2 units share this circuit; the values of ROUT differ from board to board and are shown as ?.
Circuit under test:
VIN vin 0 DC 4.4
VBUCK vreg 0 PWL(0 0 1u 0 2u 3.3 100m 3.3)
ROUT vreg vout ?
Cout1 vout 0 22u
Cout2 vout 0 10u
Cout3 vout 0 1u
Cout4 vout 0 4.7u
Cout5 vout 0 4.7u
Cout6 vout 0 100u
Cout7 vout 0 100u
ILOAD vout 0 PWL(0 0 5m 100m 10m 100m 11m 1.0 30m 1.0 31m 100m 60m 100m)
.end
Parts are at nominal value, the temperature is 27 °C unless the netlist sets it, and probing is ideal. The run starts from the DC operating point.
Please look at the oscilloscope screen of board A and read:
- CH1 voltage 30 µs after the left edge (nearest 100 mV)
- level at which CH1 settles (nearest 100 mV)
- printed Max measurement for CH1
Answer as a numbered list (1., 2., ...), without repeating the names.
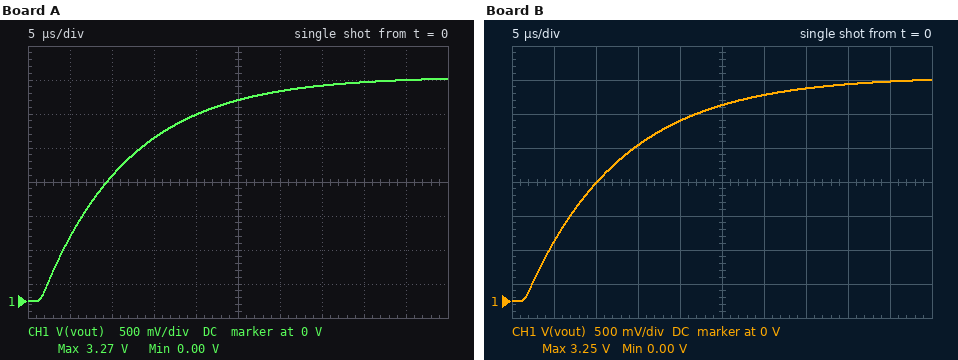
1. 3.1 V
2. 3.3 V
3. 3.27 V
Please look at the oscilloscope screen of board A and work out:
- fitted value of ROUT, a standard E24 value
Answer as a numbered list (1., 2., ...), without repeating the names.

1. 0.043 Ω
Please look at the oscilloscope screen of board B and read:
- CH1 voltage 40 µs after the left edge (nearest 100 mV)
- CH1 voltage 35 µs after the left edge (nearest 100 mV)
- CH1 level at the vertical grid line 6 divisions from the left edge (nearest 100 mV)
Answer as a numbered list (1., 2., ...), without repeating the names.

1. 3.2 V
2. 3.1 V
3. 3.0 V
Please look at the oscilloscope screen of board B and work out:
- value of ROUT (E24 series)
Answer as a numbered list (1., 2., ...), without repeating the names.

1. 0.047 Ω
